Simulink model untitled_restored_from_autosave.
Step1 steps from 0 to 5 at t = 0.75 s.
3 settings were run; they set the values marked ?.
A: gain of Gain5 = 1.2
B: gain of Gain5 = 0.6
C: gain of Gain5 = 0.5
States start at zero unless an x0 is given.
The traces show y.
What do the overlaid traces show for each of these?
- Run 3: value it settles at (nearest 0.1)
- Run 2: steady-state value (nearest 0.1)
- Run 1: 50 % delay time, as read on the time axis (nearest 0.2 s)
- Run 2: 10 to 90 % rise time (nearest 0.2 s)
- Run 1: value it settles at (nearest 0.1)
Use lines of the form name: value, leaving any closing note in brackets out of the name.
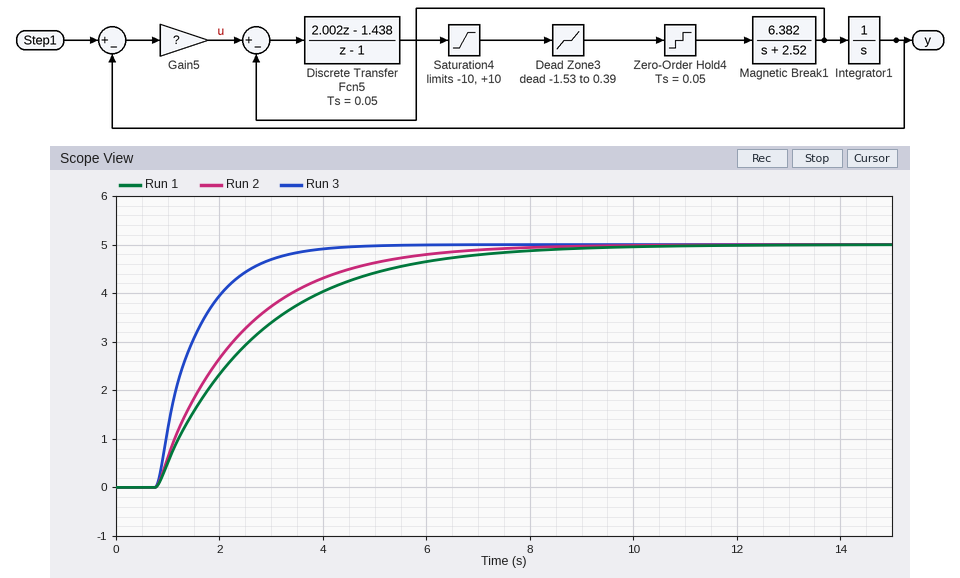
Run 3: value it settles at: 5.0
Run 2: steady-state value: 5.0
Run 1: 50 % delay time, as read on the time axis: 2.2 s
Run 2: 10 to 90 % rise time: 3.6 s
Run 1: value it settles at: 5.0
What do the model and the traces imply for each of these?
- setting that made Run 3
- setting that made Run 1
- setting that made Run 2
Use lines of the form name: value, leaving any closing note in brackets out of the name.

setting that made Run 3: A
setting that made Run 1: C
setting that made Run 2: B
